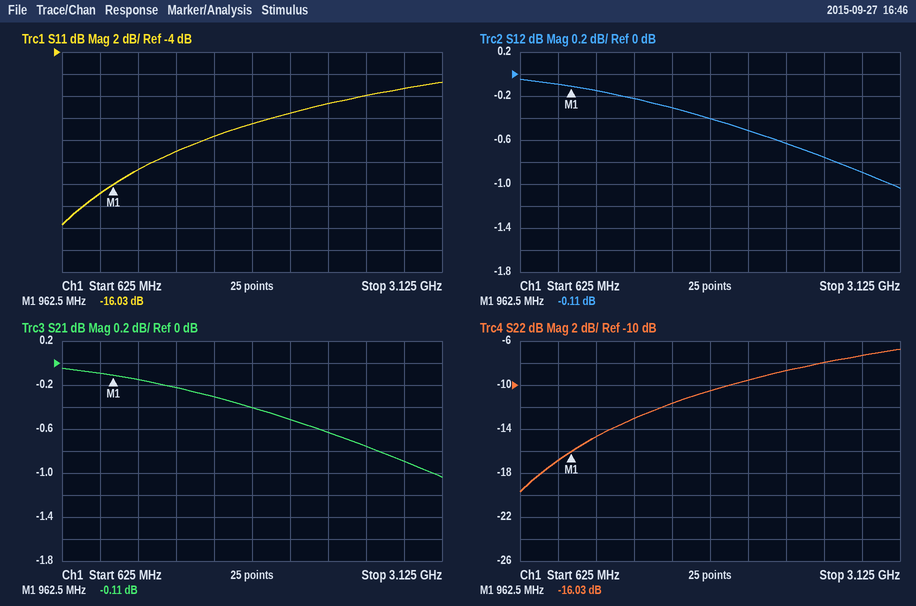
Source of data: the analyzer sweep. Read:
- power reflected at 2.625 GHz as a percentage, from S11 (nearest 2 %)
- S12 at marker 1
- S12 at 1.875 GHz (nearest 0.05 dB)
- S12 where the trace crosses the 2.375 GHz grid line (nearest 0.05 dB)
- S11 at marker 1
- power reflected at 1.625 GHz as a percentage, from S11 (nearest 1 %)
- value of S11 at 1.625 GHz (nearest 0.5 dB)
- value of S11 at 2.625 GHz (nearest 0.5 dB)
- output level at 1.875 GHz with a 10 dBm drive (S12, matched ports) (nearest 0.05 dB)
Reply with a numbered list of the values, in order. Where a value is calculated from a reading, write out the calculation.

1. 10^(-8/10) ≈ 16 %
2. -0.11 dB
3. -0.40 dB
4. -0.65 dB
5. -16.03 dB
6. 10^(-11.5/10) ≈ 7 %
7. -11.5 dB
8. -8.0 dB
9. 10 dBm + (-0.40 dB) = 9.60 dBm
